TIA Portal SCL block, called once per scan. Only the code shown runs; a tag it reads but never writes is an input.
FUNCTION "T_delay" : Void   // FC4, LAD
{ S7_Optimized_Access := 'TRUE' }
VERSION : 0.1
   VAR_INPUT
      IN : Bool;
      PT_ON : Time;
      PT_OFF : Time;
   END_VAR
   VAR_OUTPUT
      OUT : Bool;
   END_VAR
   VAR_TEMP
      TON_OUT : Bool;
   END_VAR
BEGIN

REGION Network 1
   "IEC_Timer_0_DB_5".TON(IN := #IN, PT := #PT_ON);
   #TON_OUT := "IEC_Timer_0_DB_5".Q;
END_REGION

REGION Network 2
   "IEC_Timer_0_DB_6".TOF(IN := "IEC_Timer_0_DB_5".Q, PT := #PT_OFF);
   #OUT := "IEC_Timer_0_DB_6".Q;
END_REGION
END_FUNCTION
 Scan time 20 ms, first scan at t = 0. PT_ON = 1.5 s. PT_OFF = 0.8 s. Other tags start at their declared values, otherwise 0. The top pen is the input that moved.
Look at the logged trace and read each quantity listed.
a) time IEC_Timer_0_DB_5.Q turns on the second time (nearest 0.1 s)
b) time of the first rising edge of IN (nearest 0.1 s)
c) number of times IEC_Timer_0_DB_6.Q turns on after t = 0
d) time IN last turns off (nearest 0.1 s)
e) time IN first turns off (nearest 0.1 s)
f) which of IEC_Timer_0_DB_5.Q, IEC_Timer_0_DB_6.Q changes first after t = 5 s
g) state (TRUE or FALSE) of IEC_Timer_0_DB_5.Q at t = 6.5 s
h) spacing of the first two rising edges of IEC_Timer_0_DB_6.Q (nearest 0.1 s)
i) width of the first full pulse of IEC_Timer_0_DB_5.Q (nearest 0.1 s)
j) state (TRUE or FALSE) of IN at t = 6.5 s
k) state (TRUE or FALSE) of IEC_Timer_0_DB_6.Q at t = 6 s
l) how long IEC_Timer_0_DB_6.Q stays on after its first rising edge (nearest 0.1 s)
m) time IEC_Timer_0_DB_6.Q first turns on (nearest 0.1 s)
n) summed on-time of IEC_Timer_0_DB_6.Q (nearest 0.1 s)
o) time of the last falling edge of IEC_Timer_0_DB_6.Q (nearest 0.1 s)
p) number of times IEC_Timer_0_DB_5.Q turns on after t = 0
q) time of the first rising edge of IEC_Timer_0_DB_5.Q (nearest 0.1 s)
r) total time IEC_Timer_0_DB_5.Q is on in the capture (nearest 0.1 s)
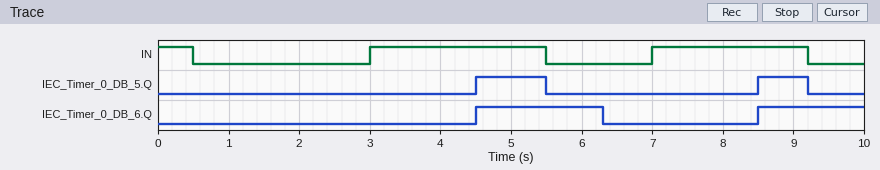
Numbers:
8.5 s
3.0 s
2
9.2 s
0.5 s
IEC_Timer_0_DB_5.Q
FALSE
4.0 s
1.0 s
FALSE
TRUE
1.8 s
4.5 s
3.3 s
6.3 s
2
4.5 s
1.7 s
